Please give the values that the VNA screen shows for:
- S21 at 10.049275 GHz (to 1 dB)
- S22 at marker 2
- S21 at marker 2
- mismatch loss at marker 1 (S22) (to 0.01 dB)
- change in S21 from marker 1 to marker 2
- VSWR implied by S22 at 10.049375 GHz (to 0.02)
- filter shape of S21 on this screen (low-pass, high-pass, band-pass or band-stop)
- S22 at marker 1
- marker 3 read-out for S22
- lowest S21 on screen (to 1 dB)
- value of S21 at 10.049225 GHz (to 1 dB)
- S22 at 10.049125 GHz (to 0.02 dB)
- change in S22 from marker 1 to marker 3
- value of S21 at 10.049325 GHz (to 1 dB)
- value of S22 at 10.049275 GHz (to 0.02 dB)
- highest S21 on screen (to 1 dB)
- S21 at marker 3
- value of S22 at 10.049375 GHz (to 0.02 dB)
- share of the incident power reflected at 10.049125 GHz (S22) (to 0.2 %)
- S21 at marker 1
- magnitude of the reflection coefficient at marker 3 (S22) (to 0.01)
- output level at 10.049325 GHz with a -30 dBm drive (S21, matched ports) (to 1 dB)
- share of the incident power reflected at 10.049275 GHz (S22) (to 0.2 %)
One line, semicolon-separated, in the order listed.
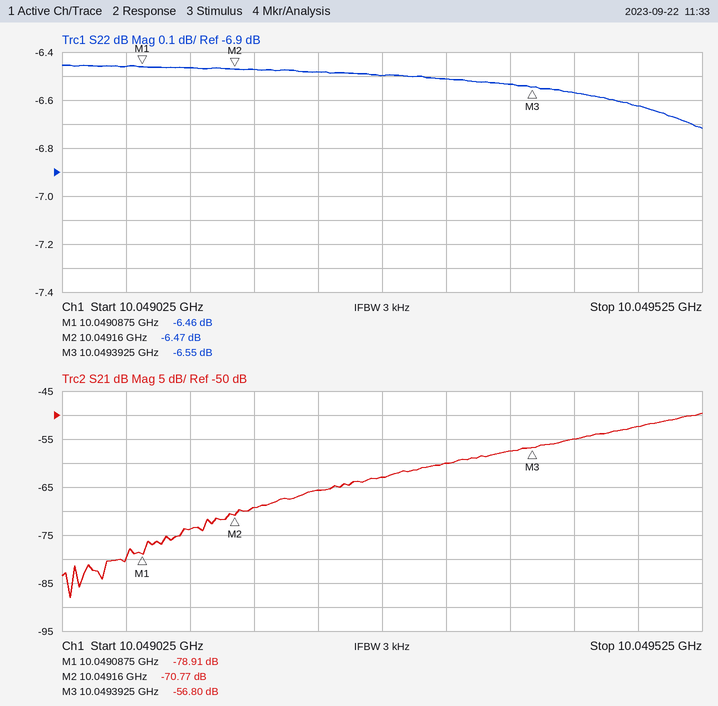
-63 dB; -6.47 dB; -70.77 dB; 1.11 dB; 8.14 dB; 2.78; high-pass; -6.46 dB; -6.55 dB; -88 dB; -66 dB; -6.46 dB; -0.09 dB; -60 dB; -6.50 dB; -50 dB; -56.80 dB; -6.54 dB; 22.6 %; -78.91 dB; 0.47; -90 dBm; 22.4 %
